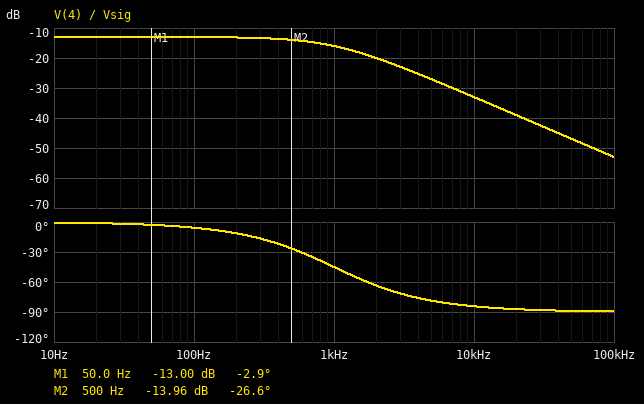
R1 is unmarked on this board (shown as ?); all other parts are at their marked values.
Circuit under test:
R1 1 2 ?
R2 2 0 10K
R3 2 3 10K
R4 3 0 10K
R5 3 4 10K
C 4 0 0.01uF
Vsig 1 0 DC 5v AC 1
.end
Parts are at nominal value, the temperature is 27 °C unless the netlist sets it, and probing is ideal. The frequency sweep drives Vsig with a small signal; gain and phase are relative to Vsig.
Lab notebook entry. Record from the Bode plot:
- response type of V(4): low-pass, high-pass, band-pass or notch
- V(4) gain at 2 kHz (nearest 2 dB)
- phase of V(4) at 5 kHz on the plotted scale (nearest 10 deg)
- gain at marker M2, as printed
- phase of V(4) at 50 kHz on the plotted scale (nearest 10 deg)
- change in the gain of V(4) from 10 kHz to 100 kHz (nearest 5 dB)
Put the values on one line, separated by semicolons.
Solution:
low-pass; -20 dB; -80 deg; -13.96 dB; -90 deg; -20 dB
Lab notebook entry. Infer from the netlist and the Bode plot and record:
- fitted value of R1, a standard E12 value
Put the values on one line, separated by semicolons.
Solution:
8.2 kΩ
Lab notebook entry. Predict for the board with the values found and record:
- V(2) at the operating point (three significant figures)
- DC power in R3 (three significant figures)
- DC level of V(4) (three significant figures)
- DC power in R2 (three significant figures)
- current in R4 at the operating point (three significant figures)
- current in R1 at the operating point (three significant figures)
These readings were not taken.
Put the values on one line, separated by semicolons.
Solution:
2.24 V; 126 µW; 1.12 V; 503 µW; 112 µA; 336 µA
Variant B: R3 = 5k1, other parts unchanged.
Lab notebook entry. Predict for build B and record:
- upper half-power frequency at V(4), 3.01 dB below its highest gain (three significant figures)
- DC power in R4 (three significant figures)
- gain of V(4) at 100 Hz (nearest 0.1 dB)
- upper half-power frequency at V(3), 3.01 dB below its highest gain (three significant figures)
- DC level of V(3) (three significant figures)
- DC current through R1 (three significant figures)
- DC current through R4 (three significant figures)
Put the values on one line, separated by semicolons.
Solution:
1.07 kHz; 196 µW; -11.1 dB; 3.39 kHz; 1.40 V; 352 µA; 140 µA
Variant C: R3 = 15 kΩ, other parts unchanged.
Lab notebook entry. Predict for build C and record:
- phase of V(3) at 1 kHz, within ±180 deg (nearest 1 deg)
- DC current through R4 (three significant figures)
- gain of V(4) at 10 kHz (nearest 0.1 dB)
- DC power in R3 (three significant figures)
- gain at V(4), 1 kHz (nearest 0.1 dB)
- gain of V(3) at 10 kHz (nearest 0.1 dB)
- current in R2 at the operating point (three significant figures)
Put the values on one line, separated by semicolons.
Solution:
-14 deg; 93.1 µA; -35.0 dB; 130 µW; -17.8 dB; -18.9 dB; 233 µA
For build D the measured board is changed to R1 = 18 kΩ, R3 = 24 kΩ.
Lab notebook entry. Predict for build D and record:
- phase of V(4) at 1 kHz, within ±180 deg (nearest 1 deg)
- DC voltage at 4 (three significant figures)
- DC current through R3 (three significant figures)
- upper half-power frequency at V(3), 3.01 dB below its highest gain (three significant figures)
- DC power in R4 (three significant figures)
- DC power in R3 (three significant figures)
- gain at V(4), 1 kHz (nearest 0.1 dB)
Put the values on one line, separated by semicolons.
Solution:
-48 deg; 442 mV; 44.2 µA; 1.54 kHz; 19.5 µW; 46.8 µW; -24.5 dB
